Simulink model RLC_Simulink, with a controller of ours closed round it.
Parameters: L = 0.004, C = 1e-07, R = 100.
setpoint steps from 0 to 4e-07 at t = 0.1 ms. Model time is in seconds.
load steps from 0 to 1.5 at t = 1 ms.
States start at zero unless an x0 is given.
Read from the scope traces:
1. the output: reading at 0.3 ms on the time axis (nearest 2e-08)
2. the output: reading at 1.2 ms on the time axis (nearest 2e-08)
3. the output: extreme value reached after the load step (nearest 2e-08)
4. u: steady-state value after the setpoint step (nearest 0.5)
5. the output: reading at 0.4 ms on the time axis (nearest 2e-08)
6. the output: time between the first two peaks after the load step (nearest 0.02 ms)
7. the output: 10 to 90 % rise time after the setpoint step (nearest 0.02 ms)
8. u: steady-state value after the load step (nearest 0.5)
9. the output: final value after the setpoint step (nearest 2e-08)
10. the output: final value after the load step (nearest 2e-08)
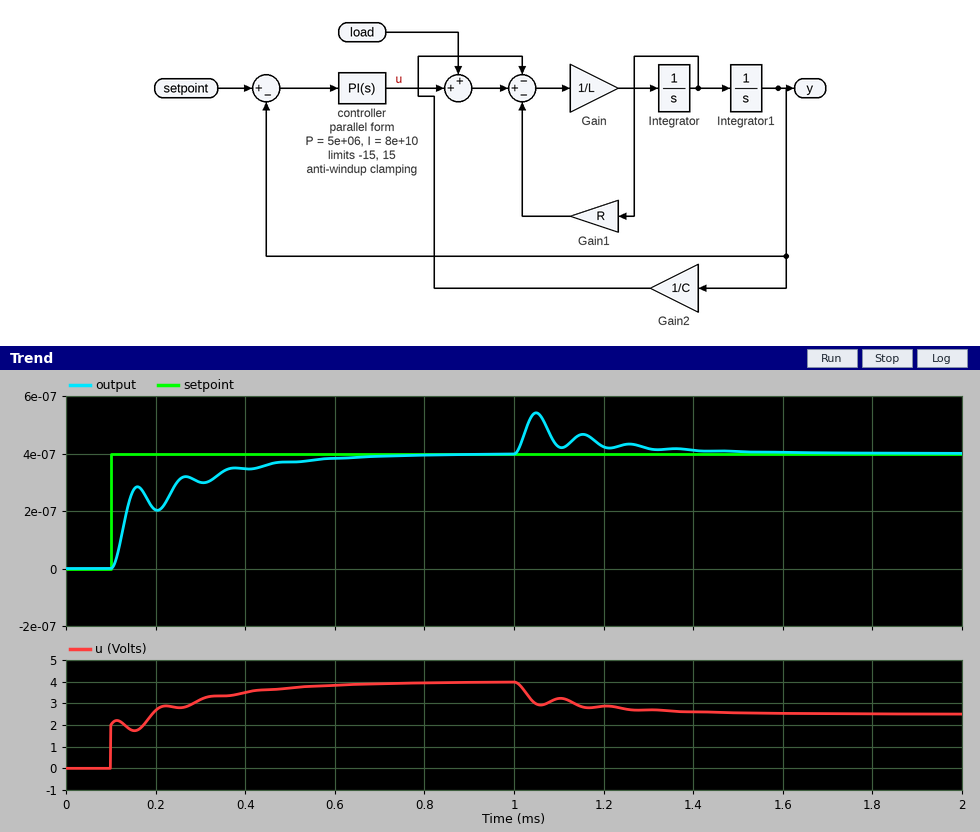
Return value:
0.00000030
0.00000042
0.00000054
4.0
0.00000034
0.10 ms
0.34 ms
2.5
0.00000040
0.00000040
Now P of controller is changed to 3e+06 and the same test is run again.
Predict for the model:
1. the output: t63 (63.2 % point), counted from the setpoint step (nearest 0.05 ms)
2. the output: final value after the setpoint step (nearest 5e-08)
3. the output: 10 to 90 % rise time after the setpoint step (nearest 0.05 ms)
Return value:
0.15 ms
0.00000040
0.30 ms
